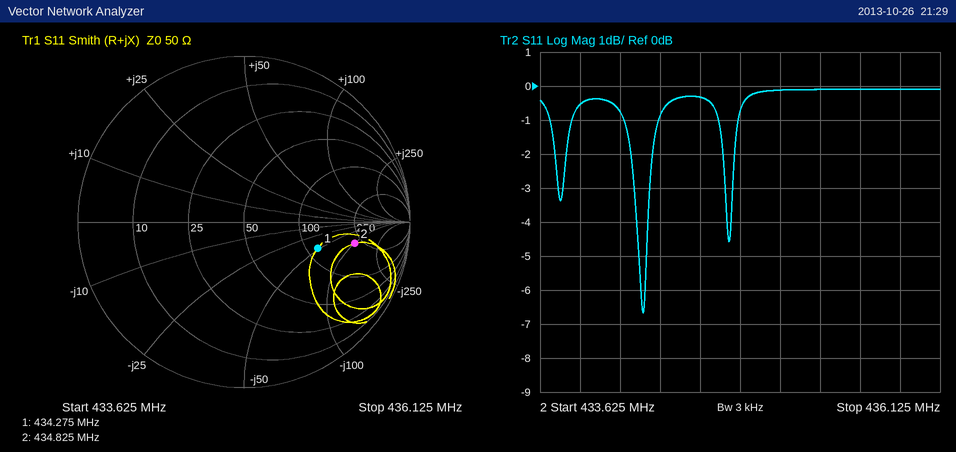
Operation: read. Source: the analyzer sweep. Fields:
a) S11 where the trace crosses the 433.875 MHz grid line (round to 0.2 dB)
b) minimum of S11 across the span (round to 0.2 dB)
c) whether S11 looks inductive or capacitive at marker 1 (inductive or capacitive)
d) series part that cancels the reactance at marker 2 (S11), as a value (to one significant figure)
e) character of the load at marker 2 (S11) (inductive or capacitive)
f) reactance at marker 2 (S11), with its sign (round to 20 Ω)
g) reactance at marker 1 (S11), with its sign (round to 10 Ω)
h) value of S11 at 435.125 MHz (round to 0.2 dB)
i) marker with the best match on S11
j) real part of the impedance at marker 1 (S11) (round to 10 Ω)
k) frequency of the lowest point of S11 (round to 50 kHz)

-0.6 dB
-6.6 dB
capacitive
40 nH
capacitive
-100 Ω
-50 Ω
-0.2 dB
marker 1
120 Ω
434.25 MHz
